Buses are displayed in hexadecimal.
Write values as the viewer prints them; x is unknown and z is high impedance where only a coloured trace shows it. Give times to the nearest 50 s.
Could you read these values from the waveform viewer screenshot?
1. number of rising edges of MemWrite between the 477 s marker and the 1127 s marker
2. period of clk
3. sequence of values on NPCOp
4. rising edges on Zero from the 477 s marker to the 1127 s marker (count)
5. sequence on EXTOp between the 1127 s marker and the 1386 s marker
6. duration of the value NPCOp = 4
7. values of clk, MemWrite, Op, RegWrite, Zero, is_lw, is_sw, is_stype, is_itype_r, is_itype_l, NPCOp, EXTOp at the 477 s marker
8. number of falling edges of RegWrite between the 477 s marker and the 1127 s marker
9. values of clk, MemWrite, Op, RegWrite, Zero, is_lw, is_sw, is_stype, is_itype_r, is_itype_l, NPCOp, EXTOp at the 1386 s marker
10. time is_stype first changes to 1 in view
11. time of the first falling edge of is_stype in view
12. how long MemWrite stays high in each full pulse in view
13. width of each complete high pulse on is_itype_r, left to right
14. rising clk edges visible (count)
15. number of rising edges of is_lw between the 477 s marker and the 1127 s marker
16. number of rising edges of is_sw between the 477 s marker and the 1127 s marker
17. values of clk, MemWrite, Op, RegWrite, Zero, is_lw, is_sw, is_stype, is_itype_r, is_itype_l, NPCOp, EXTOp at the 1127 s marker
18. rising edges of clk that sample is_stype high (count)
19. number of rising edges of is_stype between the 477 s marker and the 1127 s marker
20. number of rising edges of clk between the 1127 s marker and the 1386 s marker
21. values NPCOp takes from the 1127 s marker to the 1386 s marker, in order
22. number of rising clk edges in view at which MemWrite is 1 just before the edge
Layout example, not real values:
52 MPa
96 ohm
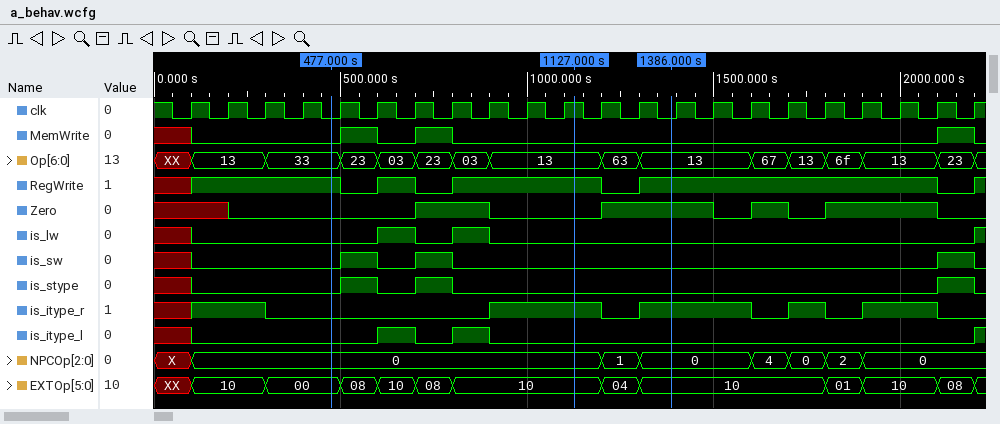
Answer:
2
100 s
X, 0, 1, 0, 4, 0, 2, 0
1
10, 04, 10
100 s
clk=0, MemWrite=0, Op=33, RegWrite=1, Zero=0, is_lw=0, is_sw=0, is_stype=0, is_itype_r=0, is_itype_l=0, NPCOp=0, EXTOp=00
2
clk=0, MemWrite=0, Op=13, RegWrite=1, Zero=1, is_lw=0, is_sw=0, is_stype=0, is_itype_r=1, is_itype_l=0, NPCOp=0, EXTOp=10
500 s
600 s
100 s, 100 s, 100 s
300 s, 300 s, 100 s, 200 s
22
2
2
clk=1, MemWrite=0, Op=13, RegWrite=1, Zero=0, is_lw=0, is_sw=0, is_stype=0, is_itype_r=1, is_itype_l=0, NPCOp=0, EXTOp=10
3
2
2
0, 1, 0
3
